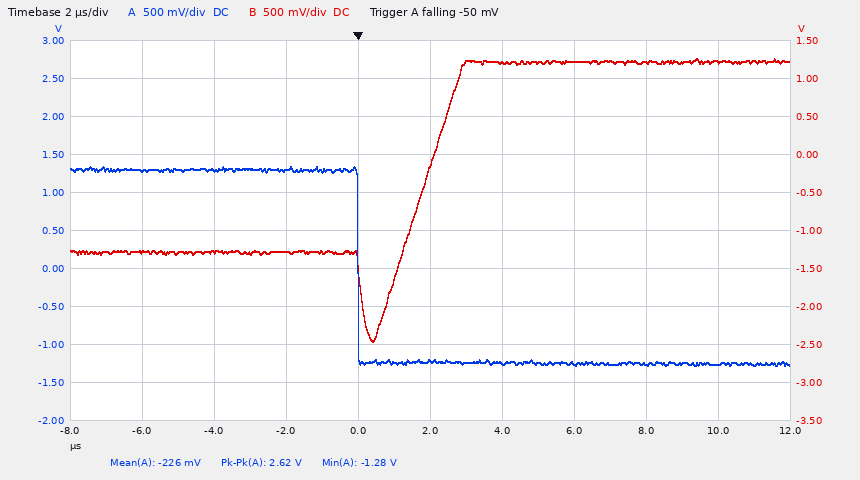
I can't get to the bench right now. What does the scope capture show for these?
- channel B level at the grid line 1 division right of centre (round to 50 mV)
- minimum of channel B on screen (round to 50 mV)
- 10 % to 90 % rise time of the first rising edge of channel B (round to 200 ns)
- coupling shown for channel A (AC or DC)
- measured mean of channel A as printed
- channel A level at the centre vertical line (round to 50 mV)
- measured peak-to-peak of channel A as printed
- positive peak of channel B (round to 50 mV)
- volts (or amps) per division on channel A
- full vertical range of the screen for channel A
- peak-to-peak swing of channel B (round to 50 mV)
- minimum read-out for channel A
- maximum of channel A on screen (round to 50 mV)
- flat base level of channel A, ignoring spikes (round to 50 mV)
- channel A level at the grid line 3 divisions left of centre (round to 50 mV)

1.20 V
-2.45 V
1.4 µs
DC
-226 mV
-1.20 V
2.62 V
1.25 V
500 mV
5 V
3.70 V
-1.28 V
1.35 V
-1.25 V
1.30 V
